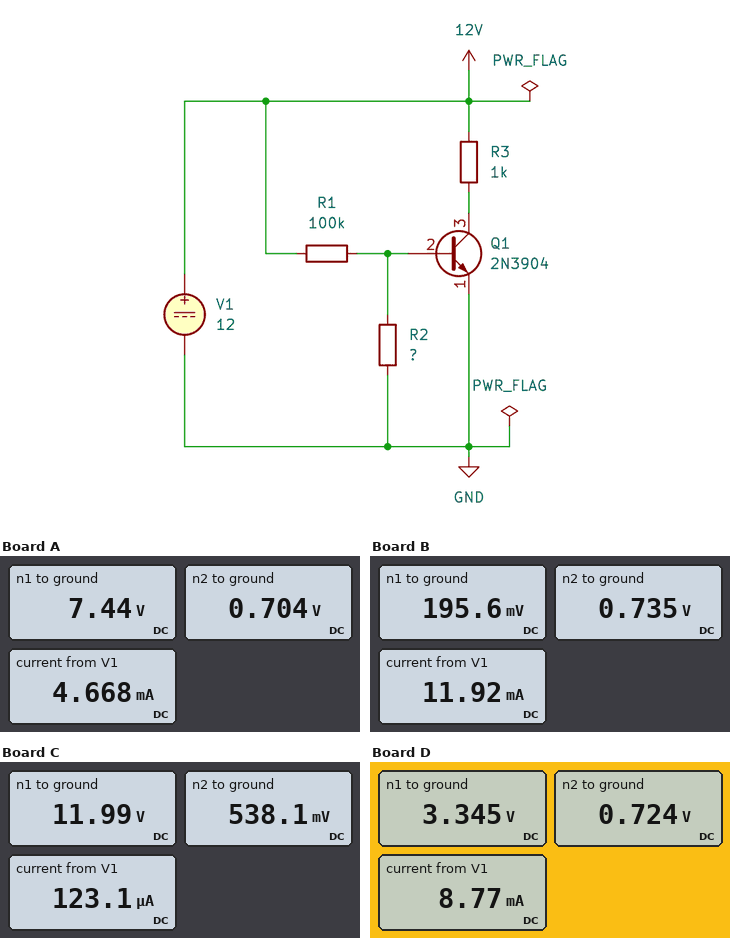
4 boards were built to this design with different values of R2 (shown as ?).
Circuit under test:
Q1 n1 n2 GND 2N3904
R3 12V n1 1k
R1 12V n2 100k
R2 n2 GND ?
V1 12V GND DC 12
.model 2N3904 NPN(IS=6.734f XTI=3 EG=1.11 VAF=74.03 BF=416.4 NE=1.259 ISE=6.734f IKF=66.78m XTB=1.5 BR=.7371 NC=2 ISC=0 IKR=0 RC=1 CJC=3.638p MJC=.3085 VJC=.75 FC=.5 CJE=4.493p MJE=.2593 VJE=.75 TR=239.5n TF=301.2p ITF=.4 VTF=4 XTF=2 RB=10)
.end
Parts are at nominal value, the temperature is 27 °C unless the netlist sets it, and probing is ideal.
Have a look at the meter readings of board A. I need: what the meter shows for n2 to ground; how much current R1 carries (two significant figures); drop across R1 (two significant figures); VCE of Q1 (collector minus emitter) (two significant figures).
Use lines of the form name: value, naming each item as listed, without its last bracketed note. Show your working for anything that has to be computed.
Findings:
what the meter shows for n2 to ground: 0.704 V
how much current R1 carries: (12 V - 704 mV) / 100 kΩ = 110 µA
drop across R1: 12 V - 704 mV = 11 V
VCE of Q1 (collector minus emitter): 7.44 V = 7.4 V
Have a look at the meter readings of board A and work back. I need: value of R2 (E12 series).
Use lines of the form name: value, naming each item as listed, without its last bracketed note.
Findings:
value of R2: 8.2 kΩ
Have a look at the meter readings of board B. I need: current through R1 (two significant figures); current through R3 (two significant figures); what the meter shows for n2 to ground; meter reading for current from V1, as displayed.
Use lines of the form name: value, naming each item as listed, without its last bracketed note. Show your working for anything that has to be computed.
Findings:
current through R1: (12 V - 735 mV) / 100 kΩ = 110 µA
current through R3: (12 V - 195.6 mV) / 1 kΩ = 12 mA
what the meter shows for n2 to ground: 0.735 V
meter reading for current from V1, as displayed: 11.92 mA
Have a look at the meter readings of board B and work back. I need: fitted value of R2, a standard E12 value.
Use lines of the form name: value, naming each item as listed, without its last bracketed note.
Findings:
fitted value of R2, a standard E12 value: 33 kΩ
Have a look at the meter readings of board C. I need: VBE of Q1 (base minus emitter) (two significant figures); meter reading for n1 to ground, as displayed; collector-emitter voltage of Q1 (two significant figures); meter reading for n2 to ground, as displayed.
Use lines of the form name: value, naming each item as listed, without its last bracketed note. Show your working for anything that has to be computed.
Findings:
VBE of Q1 (base minus emitter): 538.1 mV = 540 mV
meter reading for n1 to ground, as displayed: 11.99 V
collector-emitter voltage of Q1: 11.99 V = 12 V
meter reading for n2 to ground, as displayed: 538.1 mV
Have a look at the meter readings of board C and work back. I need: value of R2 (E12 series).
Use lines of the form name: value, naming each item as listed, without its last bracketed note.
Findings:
value of R2: 4.7 kΩ
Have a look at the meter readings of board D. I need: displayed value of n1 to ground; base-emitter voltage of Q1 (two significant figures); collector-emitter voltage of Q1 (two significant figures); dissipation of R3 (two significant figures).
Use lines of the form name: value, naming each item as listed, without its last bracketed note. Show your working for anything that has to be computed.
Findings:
displayed value of n1 to ground: 3.345 V
base-emitter voltage of Q1: 724 mV = 720 mV
collector-emitter voltage of Q1: 3.345 V = 3.3 V
dissipation of R3: (12 V - 3.345 V)^2 / 1 kΩ = 75 mW
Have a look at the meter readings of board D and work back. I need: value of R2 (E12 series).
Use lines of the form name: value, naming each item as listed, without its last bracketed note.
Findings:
value of R2: 12 kΩ
